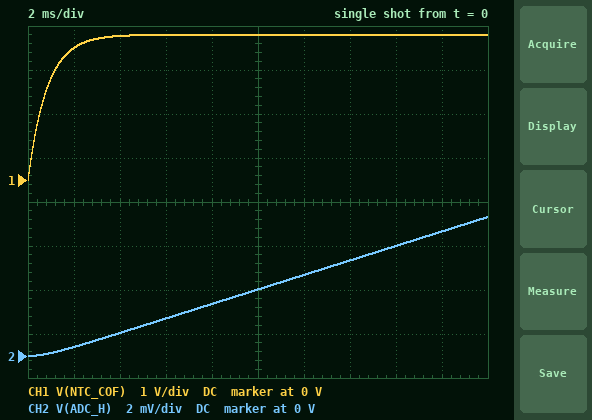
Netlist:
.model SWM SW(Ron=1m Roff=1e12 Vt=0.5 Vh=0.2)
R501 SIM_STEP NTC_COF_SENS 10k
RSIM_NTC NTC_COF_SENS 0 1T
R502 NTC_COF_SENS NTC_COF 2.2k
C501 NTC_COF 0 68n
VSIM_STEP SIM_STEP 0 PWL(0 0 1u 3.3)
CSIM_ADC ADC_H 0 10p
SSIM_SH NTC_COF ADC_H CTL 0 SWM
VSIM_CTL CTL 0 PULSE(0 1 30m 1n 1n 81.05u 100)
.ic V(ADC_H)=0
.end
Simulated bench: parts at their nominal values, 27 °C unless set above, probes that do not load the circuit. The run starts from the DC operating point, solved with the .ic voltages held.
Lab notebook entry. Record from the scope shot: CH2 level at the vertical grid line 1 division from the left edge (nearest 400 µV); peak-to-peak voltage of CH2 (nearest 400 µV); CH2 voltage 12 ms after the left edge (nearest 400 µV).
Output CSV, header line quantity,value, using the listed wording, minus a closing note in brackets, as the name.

quantity,value
CH2 level at the vertical grid line 1 division from the left edge,400 µV
peak-to-peak voltage of CH2,6.4 mV
CH2 voltage 12 ms after the left edge,3.6 mV
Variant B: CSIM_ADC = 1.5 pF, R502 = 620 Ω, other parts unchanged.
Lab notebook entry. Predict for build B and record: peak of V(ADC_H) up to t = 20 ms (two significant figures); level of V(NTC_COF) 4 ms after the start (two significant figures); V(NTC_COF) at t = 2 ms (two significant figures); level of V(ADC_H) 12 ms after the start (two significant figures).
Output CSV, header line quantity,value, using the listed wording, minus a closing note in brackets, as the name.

quantity,value
peak of V(ADC_H) up to t = 20 ms,42 mV
level of V(NTC_COF) 4 ms after the start,3.3 V
V(NTC_COF) at t = 2 ms,3.1 V
level of V(ADC_H) 12 ms after the start,25 mV
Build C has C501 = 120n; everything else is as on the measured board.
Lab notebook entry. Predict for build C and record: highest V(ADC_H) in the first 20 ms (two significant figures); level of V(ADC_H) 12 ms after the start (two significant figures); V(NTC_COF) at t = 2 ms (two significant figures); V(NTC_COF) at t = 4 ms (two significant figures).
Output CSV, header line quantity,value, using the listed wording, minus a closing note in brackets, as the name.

quantity,value
highest V(ADC_H) in the first 20 ms,6.1 mV
level of V(ADC_H) 12 ms after the start,3.5 mV
V(NTC_COF) at t = 2 ms,2.5 V
V(NTC_COF) at t = 4 ms,3.1 V
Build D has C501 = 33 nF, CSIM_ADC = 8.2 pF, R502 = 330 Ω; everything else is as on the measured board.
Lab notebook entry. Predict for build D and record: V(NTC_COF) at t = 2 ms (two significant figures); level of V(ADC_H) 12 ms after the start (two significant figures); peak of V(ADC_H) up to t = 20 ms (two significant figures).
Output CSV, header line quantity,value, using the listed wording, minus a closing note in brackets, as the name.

quantity,value
V(NTC_COF) at t = 2 ms,3.3 V
level of V(ADC_H) 12 ms after the start,4.7 mV
peak of V(ADC_H) up to t = 20 ms,7.9 mV
